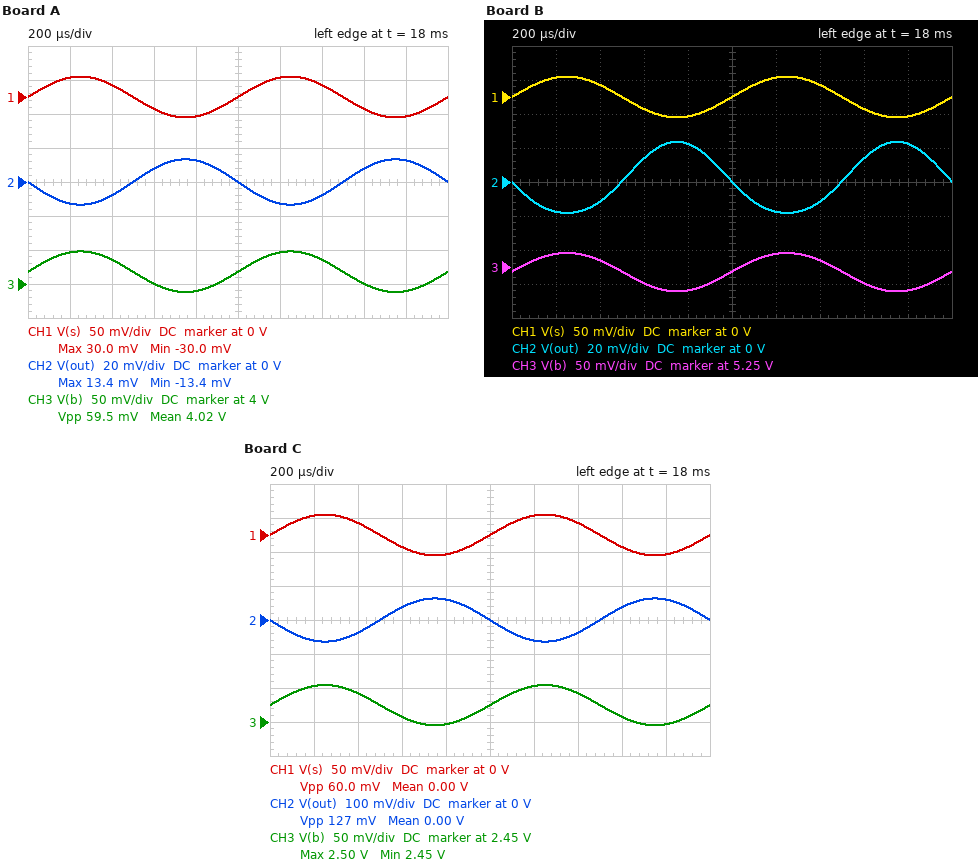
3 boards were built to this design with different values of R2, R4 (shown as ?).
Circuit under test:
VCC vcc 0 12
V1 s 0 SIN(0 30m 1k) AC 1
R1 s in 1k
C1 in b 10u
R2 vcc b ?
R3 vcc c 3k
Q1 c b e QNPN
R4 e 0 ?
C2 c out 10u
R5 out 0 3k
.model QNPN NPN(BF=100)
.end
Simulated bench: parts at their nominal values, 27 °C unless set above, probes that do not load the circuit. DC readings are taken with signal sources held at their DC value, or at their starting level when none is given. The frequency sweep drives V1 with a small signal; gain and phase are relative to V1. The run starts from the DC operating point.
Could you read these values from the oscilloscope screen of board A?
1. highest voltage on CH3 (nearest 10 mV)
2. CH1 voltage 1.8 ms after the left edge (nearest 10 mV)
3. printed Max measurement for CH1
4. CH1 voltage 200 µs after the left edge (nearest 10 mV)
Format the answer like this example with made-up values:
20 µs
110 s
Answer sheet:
4.05 V
-30 mV
30.0 mV
30 mV
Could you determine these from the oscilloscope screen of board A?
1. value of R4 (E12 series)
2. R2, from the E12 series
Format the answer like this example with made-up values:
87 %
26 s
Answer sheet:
3.3 kΩ
820 kΩ
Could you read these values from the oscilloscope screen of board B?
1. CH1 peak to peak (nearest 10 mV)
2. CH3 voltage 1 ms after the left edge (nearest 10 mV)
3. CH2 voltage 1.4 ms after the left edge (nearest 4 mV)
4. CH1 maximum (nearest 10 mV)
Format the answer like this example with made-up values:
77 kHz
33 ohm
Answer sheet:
60 mV
5.24 V
-12 mV
30 mV
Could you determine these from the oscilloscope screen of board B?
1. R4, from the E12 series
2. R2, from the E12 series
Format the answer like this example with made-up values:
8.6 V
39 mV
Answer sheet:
1.8 kΩ
270 kΩ
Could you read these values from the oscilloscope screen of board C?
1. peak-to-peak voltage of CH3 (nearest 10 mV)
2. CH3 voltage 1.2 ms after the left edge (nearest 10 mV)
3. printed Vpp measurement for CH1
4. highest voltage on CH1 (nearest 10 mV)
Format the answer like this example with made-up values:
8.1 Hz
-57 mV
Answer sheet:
60 mV
2.50 V
60.0 mV
30 mV
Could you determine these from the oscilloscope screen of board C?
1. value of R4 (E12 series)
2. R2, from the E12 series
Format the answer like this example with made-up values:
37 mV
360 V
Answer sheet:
680 Ω
390 kΩ
